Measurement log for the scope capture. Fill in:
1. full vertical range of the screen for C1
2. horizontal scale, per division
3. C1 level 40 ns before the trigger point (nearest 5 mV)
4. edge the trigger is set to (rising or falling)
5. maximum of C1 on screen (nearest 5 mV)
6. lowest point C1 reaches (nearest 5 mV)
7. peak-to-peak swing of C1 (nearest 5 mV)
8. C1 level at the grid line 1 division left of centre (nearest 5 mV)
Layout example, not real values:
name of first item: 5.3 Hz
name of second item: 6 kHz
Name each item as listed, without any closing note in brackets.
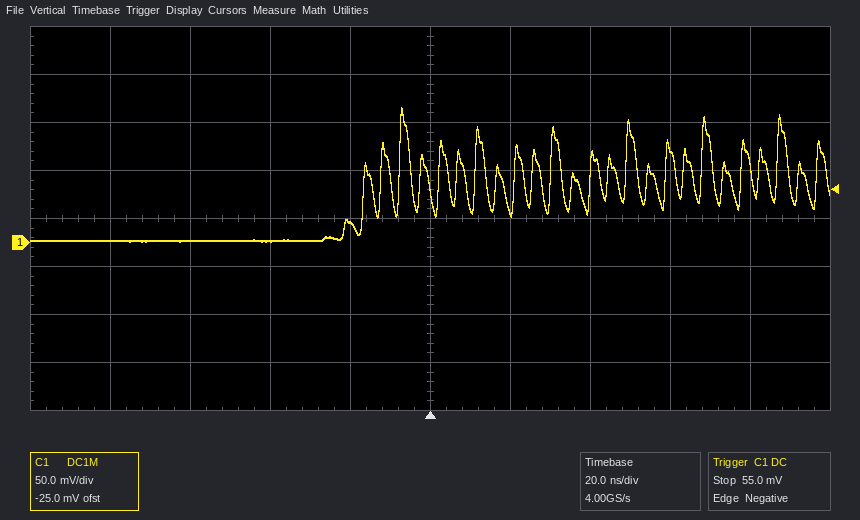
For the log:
full vertical range of the screen for C1: 400 mV
horizontal scale, per division: 20 ns
C1 level 40 ns before the trigger point: 0 mV
edge the trigger is set to: falling
maximum of C1 on screen: 140 mV
lowest point C1 reaches: 0 mV
peak-to-peak swing of C1: 140 mV
C1 level at the grid line 1 division left of centre: 20 mV
